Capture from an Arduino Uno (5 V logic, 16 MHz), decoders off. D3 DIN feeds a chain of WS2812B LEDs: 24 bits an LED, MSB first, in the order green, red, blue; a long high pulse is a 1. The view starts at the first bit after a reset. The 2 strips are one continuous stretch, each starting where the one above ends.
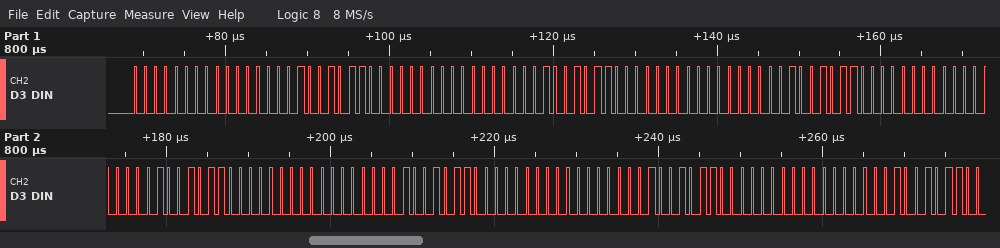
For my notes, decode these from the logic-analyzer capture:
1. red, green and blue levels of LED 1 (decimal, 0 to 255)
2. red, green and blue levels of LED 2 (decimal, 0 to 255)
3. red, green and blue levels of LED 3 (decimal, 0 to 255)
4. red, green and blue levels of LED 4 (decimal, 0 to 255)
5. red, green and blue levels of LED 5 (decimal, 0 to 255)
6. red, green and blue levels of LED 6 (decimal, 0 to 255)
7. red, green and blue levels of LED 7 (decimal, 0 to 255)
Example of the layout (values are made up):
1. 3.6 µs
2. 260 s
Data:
1. 0, 0, 150
2. 0, 0, 150
3. 0, 0, 150
4. 0, 0, 150
5. 0, 0, 150
6. 0, 0, 150
7. 0, 0, 150
